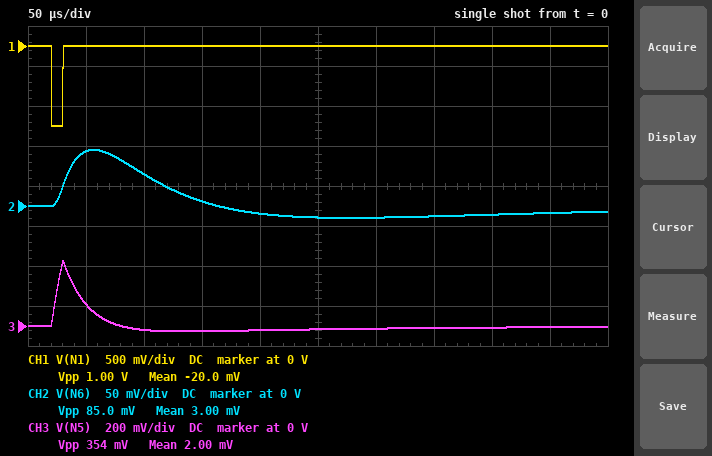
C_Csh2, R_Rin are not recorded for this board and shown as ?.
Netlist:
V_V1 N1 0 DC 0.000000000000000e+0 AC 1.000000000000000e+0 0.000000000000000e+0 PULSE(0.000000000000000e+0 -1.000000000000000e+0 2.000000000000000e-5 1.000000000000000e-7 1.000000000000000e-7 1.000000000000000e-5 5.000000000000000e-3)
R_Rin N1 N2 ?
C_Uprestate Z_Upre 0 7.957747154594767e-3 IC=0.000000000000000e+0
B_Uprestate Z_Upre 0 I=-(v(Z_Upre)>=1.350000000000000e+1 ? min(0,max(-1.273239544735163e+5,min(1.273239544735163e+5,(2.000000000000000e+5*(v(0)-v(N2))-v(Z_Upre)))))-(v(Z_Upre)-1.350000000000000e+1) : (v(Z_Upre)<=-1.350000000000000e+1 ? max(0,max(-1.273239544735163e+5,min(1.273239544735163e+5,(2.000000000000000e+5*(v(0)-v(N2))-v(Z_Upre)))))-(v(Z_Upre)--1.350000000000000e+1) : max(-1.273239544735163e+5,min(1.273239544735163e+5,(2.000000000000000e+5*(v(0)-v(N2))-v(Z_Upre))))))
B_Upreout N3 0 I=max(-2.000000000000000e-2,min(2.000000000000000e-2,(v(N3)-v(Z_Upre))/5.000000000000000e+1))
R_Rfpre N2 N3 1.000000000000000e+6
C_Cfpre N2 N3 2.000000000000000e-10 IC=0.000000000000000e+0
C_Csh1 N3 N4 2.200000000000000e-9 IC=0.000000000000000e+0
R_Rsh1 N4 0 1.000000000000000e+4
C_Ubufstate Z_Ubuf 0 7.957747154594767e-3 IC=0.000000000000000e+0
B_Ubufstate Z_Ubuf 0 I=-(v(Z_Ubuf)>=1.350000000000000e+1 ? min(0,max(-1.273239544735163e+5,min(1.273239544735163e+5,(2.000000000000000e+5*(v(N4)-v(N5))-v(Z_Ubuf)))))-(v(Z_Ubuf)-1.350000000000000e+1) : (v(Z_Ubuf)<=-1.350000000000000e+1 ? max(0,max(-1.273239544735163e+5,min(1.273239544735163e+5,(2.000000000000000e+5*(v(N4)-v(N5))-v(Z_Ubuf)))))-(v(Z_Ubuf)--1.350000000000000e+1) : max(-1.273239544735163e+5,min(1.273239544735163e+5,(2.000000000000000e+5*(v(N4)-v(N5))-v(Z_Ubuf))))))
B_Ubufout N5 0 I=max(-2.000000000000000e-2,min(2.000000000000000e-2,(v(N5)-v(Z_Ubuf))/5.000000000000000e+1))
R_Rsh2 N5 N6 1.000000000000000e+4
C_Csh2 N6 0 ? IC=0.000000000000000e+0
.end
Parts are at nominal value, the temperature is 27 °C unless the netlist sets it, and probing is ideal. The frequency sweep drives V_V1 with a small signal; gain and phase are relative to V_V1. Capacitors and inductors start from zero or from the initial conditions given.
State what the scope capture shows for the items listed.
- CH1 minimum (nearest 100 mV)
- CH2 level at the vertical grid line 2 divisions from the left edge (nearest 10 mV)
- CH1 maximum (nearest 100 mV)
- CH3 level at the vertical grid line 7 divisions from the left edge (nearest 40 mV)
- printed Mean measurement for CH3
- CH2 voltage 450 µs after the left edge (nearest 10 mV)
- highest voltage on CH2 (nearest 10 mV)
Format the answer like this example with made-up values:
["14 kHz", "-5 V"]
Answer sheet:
["-1.0 V", "40 mV", "0 V", "0 V", "2.00 mV", "-10 mV", "70 mV"]
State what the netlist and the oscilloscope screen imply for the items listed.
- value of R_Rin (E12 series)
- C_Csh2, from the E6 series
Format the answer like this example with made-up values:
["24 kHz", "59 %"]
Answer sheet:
["120 kΩ", "6.8 nF"]
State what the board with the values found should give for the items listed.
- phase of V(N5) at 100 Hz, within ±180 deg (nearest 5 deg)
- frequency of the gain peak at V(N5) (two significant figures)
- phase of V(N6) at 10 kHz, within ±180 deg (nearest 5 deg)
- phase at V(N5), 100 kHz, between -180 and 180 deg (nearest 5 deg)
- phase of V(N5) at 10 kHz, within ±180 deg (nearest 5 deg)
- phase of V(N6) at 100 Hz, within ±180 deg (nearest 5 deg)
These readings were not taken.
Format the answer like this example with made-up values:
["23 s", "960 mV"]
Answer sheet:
["-100 deg", "2.4 kHz", "55 deg", "90 deg", "130 deg", "-100 deg"]
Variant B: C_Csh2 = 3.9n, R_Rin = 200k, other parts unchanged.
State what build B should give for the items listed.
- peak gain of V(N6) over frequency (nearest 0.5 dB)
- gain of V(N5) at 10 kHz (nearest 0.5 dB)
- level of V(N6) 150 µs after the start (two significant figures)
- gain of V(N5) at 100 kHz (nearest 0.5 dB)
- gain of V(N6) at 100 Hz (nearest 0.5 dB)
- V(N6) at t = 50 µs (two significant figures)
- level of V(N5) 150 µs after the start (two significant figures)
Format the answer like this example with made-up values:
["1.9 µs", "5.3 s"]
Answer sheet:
["-7.0 dB", "-10.0 dB", "-5.4 mV", "-28.0 dB", "-23.5 dB", "61 mV", "-16 mV"]
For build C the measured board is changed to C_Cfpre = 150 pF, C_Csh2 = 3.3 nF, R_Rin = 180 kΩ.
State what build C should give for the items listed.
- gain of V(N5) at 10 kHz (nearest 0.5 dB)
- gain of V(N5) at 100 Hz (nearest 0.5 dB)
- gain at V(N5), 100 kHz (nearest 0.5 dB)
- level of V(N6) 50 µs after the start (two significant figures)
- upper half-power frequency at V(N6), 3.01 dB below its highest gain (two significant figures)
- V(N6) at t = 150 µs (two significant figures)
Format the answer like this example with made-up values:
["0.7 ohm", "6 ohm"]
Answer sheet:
["-6.5 dB", "-22.5 dB", "-24.5 dB", "98 mV", "5.0 kHz", "-17 mV"]
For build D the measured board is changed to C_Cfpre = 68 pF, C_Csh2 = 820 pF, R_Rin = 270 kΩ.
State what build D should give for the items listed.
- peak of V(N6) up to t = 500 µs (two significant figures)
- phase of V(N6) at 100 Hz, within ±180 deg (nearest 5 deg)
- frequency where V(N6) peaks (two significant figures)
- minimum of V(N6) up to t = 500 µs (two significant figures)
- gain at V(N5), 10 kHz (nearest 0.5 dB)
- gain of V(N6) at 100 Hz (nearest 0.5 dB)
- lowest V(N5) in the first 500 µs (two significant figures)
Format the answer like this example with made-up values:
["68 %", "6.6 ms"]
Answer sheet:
["260 mV", "-95 deg", "3.9 kHz", "-58 mV", "-3.5 dB", "-26.0 dB", "-60 mV"]
